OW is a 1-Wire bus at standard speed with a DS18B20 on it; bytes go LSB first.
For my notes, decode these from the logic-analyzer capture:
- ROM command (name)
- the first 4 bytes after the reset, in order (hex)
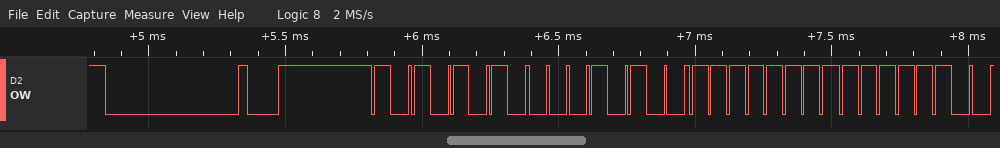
Match ROM
55 28 FF 3F
